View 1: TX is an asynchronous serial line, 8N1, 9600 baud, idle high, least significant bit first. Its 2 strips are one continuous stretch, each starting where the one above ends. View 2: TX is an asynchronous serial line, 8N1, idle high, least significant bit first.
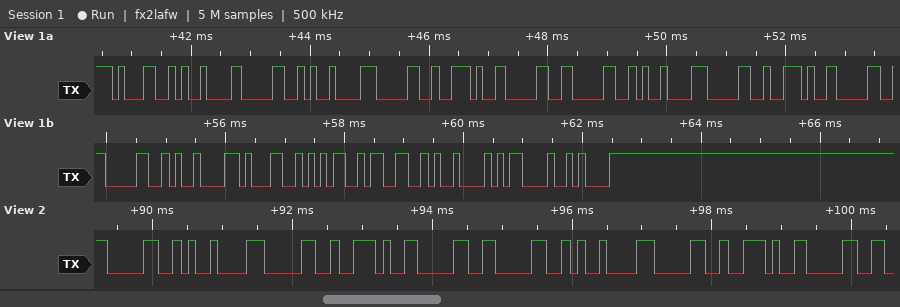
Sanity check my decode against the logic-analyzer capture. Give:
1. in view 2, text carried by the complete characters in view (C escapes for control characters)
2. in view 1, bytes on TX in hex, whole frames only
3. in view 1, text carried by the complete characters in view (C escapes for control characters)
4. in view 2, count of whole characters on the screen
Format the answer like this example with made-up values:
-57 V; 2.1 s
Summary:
"0\t0.00\t0.0"; 0x31 0x09 0x30 0x09 0x30 0x2E 0x30 0x30 0x09 0x30 0x2E 0x30 0x30 0x09 0x31 0x35 0x33 0x09 0x0D 0x0A; "1\t0\t0.00\t0.00\t153\t\r\n"; 10
